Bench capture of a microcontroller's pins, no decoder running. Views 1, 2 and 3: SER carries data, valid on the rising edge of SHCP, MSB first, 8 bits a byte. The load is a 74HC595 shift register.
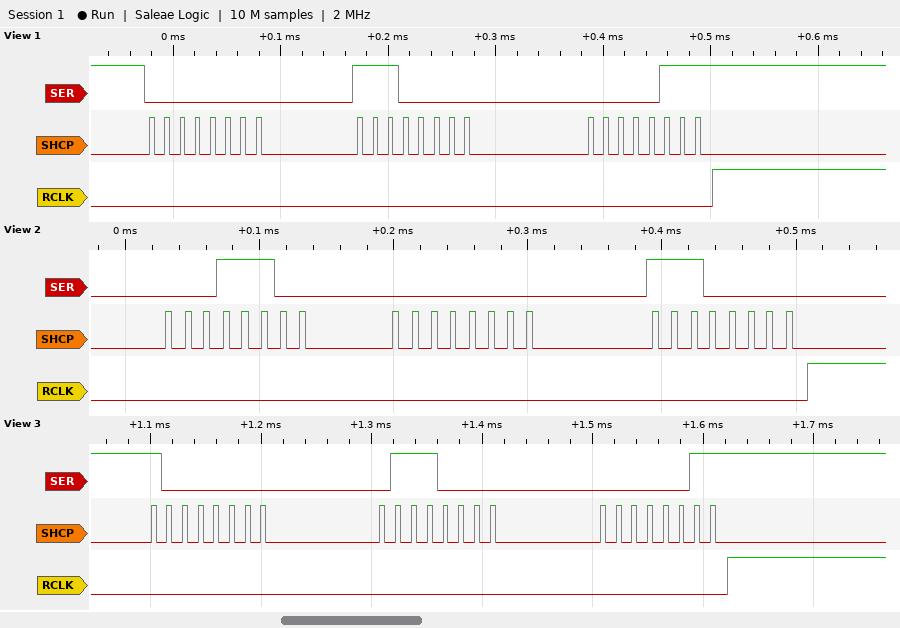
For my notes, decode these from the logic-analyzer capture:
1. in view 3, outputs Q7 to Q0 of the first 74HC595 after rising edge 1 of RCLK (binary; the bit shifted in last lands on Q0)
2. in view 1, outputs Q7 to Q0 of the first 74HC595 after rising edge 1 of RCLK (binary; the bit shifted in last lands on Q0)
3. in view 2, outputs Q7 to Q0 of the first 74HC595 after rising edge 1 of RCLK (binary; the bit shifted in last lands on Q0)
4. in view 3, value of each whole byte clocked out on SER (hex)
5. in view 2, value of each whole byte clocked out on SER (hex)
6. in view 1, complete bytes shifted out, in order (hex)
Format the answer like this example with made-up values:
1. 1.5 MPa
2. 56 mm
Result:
1. 00000011
2. 00000111
3. 11100000
4. 80 70 03
5. 1C 00 E0
6. 00 E0 07
